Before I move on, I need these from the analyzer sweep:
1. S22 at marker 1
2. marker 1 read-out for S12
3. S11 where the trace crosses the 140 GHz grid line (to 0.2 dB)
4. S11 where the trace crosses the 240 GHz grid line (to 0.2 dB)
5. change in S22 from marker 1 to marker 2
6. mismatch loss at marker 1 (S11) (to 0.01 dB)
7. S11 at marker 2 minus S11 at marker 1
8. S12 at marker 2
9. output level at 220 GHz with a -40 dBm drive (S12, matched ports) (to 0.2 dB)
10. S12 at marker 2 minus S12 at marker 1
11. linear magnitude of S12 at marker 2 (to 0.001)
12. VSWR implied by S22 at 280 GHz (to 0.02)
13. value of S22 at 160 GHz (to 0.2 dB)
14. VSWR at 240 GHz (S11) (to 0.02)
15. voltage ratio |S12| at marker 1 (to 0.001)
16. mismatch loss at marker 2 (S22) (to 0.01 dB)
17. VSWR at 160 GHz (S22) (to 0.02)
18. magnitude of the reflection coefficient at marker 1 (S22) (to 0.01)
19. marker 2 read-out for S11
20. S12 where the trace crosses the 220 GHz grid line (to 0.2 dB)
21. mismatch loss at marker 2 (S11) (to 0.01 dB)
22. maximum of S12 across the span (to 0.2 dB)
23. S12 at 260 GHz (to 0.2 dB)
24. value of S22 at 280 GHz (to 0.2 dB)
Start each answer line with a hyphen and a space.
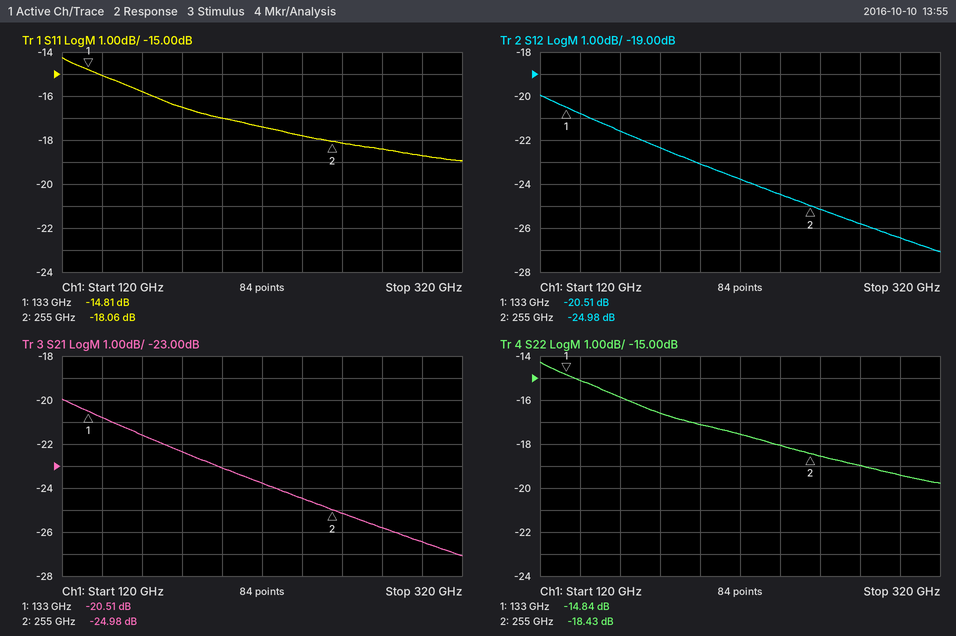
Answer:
- -14.84 dB
- -20.51 dB
- -15.0 dB
- -17.8 dB
- -3.59 dB
- 0.15 dB
- -3.25 dB
- -24.98 dB
- -63.8 dBm
- -4.47 dB
- 0.056
- 1.26
- -15.8 dB
- 1.30
- 0.094
- 0.06 dB
- 1.38
- 0.18
- -18.06 dB
- -23.8 dB
- 0.07 dB
- -20.0 dB
- -25.2 dB
- -19.0 dB
